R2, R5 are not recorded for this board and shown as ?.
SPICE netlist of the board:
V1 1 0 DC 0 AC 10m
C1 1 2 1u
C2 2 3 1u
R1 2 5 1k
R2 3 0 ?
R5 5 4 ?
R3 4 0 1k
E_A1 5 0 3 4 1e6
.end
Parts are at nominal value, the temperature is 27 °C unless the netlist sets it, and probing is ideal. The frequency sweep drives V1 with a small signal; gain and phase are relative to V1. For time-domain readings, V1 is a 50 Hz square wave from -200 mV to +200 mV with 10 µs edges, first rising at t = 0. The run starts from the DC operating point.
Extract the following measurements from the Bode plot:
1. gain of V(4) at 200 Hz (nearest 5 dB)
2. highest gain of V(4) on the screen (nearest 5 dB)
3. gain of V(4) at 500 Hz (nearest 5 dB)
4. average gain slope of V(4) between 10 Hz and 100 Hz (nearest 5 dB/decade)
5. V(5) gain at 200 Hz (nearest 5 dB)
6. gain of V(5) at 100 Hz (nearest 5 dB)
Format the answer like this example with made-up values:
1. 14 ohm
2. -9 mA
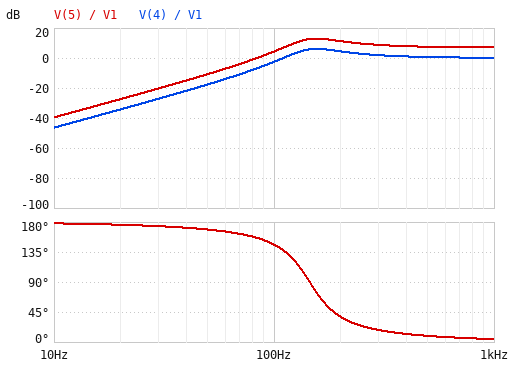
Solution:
1. 5 dB
2. 5 dB
3. 0 dB
4. 45 dB/decade
5. 10 dB
6. 5 dB
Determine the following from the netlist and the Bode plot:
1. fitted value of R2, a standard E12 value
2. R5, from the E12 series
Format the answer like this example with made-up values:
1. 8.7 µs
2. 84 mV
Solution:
1. 1.2 kΩ
2. 1.2 kΩ
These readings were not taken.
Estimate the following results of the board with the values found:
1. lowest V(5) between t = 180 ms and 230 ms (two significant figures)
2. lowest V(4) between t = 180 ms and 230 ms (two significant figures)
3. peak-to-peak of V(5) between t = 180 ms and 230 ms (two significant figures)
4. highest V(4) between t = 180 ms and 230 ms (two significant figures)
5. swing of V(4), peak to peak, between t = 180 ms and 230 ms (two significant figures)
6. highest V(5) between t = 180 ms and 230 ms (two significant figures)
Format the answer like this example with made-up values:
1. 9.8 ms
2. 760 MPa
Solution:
1. -970 mV
2. -440 mV
3. 1.9 V
4. 440 mV
5. 880 mV
6. 970 mV
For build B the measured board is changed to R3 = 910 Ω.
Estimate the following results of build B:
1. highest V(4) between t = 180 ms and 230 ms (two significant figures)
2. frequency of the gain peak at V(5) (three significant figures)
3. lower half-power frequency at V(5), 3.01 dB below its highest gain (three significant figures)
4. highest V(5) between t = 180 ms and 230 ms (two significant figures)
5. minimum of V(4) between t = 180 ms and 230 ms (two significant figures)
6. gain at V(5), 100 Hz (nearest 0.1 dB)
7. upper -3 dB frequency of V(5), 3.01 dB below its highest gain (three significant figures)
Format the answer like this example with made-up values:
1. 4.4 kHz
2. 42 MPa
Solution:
1. 480 mV
2. 151 Hz
3. 127 Hz
4. 1.1 V
5. -480 mV
6. 5.4 dB
7. 195 Hz
